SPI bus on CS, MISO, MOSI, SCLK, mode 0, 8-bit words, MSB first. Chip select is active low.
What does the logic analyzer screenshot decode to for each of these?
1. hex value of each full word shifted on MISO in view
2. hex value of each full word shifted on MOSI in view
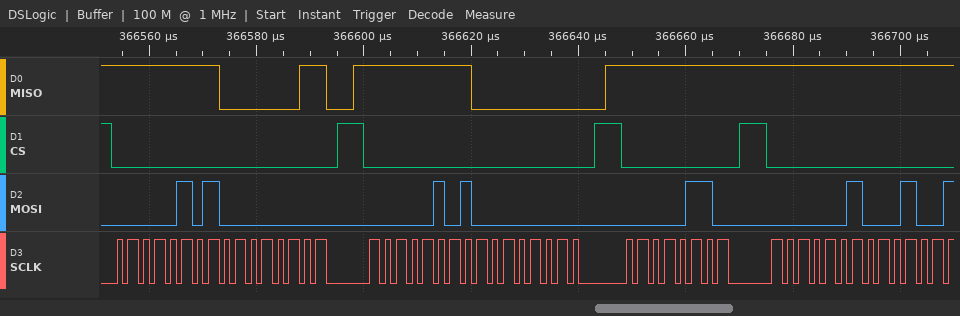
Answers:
FF, 03, FF, 00, FF, FF
05, 00, 05, 00, 06, 02
